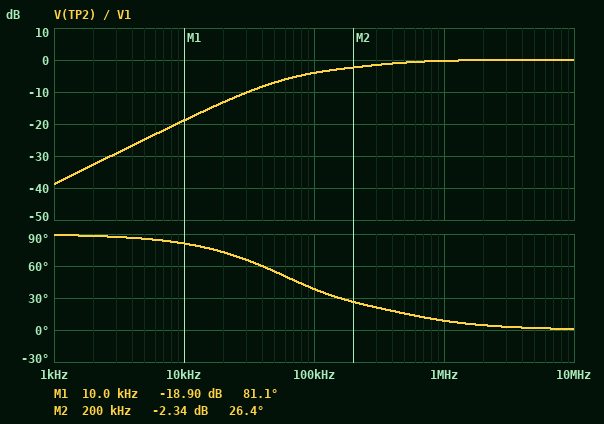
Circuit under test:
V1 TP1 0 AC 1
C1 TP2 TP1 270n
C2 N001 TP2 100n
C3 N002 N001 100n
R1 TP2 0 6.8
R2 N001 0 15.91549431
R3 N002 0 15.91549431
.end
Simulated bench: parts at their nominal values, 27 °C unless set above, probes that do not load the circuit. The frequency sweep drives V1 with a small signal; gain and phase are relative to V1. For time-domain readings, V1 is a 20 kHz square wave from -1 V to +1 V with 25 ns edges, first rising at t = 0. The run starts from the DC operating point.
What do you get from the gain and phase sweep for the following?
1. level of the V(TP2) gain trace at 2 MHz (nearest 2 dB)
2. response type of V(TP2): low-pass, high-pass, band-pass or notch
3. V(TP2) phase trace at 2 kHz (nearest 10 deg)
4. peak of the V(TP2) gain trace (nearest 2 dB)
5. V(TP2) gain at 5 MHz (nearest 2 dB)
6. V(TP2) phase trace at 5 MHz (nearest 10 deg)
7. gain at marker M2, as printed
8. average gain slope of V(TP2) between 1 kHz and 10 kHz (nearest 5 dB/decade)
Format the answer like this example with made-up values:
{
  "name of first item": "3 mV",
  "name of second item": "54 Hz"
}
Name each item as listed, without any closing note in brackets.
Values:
{
  "level of the V(TP2) gain trace at 2 MHz": "0 dB",
  "response type of V(TP2): low-pass, high-pass, band-pass or notch": "high-pass",
  "V(TP2) phase trace at 2 kHz": "90 deg",
  "peak of the V(TP2) gain trace": "0 dB",
  "V(TP2) gain at 5 MHz": "0 dB",
  "V(TP2) phase trace at 5 MHz": "0 deg",
  "gain at marker M2, as printed": "-2.34 dB",
  "average gain slope of V(TP2) between 1 kHz and 10 kHz": "20 dB/decade"
}
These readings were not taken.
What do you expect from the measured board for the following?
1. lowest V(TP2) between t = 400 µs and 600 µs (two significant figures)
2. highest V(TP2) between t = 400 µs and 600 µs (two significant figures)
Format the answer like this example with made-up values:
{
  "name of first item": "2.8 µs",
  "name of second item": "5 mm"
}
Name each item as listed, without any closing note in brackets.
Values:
{
  "lowest V(TP2) between t = 400 µs and 600 µs": "-2.0 V",
  "highest V(TP2) between t = 400 µs and 600 µs": "2.0 V"
}
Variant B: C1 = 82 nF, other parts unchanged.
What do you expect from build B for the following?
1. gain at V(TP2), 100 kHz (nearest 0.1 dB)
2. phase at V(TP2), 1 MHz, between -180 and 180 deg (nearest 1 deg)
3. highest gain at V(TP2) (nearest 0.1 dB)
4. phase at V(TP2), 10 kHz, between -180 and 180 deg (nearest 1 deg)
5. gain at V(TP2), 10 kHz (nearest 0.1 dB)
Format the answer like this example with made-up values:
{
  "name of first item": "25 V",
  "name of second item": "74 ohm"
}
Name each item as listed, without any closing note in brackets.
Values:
{
  "gain at V(TP2), 100 kHz": "-11.4 dB",
  "phase at V(TP2), 1 MHz, between -180 and 180 deg": "26 deg",
  "highest gain at V(TP2)": "0 dB",
  "phase at V(TP2), 10 kHz, between -180 and 180 deg": "86 deg",
  "gain at V(TP2), 10 kHz": "-29.2 dB"
}
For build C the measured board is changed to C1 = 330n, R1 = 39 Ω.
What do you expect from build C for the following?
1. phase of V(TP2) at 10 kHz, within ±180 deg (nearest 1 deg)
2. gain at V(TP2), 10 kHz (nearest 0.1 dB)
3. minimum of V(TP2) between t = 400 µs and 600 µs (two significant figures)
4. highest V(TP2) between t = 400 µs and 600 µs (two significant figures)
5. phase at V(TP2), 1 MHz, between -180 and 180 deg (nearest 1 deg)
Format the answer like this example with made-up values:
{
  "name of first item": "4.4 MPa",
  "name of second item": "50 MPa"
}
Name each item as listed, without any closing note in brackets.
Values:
{
  "phase of V(TP2) at 10 kHz, within ±180 deg": "44 deg",
  "gain at V(TP2), 10 kHz": "-5.2 dB",
  "minimum of V(TP2) between t = 400 µs and 600 µs": "-1.7 V",
  "highest V(TP2) between t = 400 µs and 600 µs": "1.7 V",
  "phase at V(TP2), 1 MHz, between -180 and 180 deg": "4 deg"
}
